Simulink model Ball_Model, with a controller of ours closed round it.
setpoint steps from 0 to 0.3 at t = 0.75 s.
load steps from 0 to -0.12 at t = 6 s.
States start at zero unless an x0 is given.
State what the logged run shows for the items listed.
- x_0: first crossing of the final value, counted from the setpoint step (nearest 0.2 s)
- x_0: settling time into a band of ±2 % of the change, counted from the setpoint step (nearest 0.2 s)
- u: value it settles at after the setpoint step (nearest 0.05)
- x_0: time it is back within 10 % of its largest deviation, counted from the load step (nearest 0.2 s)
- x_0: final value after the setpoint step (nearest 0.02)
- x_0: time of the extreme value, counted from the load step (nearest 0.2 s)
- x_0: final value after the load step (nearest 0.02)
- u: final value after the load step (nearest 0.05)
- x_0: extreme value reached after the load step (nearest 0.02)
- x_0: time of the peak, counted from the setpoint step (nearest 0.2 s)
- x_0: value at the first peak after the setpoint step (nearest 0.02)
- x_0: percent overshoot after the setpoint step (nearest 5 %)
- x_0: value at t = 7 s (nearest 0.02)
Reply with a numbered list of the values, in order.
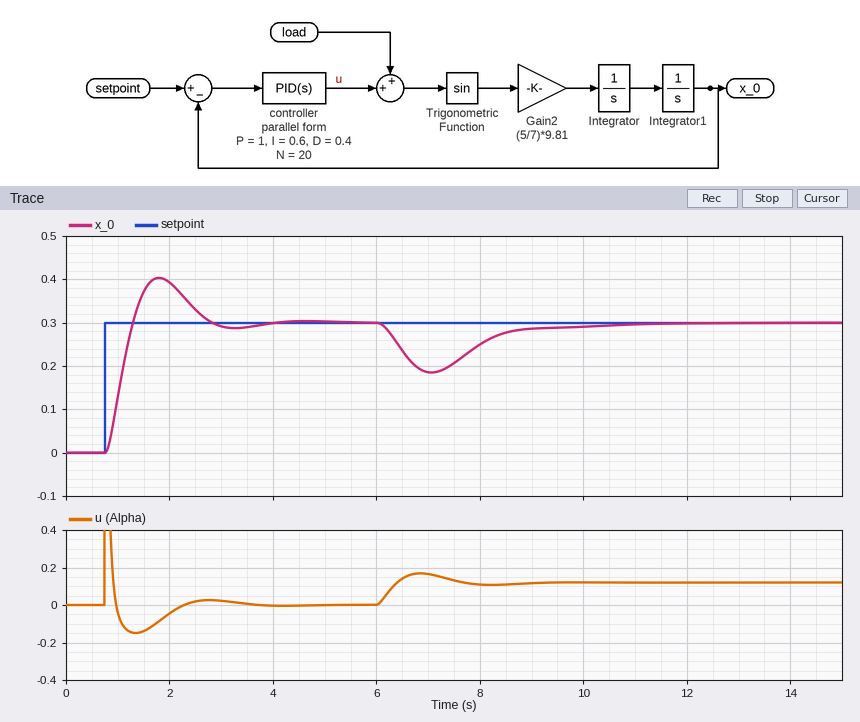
1. 0.6 s
2. 3.0 s
3. 0.00
4. 3.6 s
5. 0.30
6. 1.0 s
7. 0.30
8. 0.10
9. 0.18
10. 1.0 s
11. 0.40
12. 35 %
13. 0.18
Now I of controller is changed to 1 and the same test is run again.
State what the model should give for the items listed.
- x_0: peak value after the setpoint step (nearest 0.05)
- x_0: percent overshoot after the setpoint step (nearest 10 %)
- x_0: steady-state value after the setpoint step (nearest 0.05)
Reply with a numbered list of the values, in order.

1. 0.45
2. 40 %
3. 0.30
